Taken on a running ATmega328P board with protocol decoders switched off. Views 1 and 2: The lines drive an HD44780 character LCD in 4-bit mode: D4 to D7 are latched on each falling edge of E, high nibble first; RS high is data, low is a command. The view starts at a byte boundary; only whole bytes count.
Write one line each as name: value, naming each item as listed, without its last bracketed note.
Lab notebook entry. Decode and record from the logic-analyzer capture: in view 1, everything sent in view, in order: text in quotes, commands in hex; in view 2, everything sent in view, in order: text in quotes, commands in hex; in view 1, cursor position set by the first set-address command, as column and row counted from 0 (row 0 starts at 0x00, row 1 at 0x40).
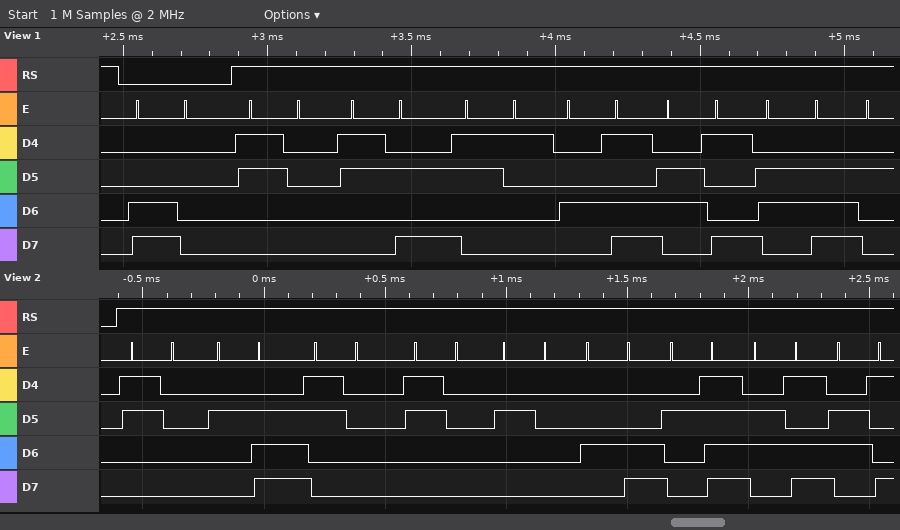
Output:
in view 1, everything sent in view, in order: text in quotes, commands in hex: 0xC0 "0:1Min"
in view 2, everything sent in view, in order: text in quotes, commands in hex: "0.00 L/mi"
in view 1, cursor position set by the first set-address command, as column and row counted from 0: column 0, row 1
